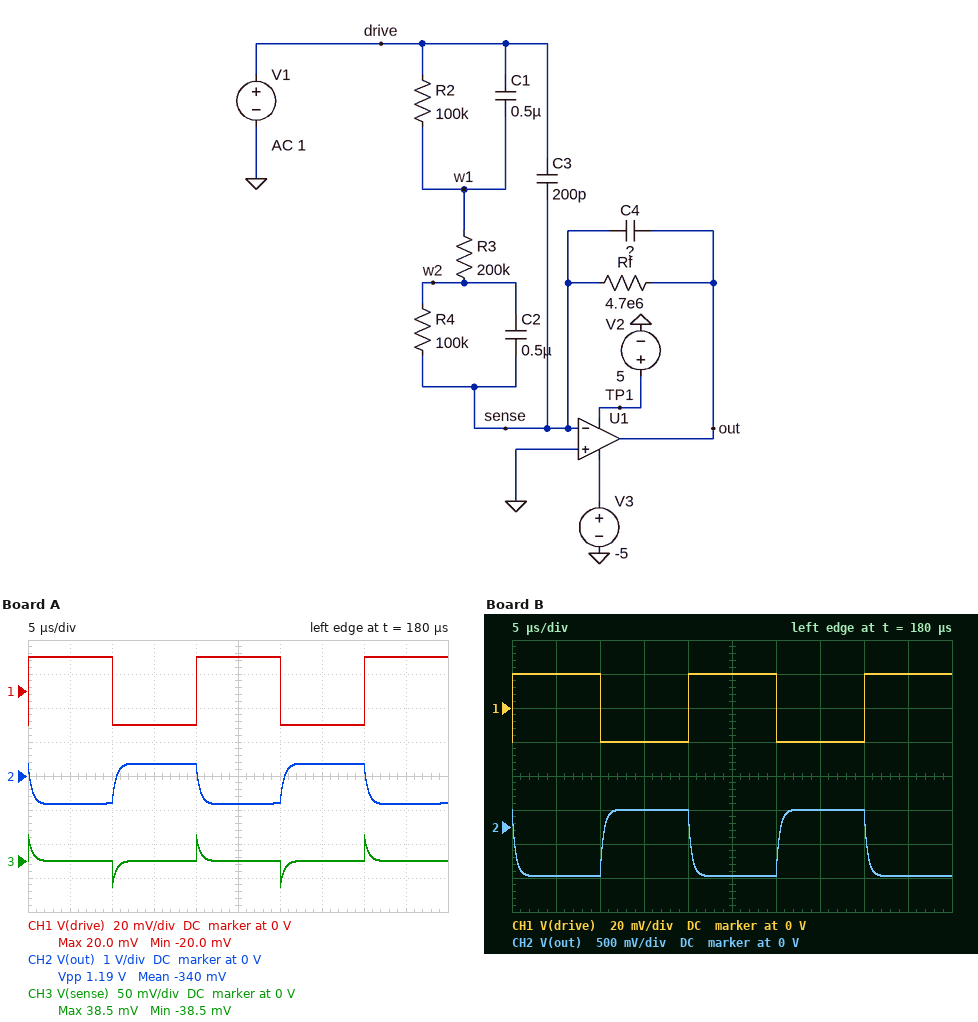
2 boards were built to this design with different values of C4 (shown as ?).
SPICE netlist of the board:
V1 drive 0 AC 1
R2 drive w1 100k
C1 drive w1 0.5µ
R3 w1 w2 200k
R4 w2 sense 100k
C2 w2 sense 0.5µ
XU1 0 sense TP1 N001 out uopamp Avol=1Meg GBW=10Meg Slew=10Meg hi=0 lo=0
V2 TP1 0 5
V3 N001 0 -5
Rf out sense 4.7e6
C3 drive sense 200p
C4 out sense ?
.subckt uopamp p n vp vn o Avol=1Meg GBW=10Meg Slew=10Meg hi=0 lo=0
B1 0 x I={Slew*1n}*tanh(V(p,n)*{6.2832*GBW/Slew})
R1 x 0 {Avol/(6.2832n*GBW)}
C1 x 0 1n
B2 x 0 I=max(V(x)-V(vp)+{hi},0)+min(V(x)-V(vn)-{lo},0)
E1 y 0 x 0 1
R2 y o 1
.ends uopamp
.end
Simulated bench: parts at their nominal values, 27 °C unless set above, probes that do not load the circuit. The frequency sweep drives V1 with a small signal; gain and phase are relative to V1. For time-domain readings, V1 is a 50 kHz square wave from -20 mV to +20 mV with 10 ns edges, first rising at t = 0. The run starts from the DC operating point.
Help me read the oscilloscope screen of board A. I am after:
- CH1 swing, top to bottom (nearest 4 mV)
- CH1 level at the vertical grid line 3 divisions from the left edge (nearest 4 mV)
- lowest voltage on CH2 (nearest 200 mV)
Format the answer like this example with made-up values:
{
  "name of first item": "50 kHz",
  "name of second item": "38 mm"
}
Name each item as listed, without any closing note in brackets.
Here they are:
{
  "CH1 swing, top to bottom": "40 mV",
  "CH1 level at the vertical grid line 3 divisions from the left edge": "-20 mV",
  "lowest voltage on CH2": "-800 mV"
}
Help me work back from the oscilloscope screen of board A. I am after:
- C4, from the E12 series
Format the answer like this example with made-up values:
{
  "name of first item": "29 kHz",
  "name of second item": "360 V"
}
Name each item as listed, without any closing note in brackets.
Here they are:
{
  "C4, from the E12 series": "6.8 pF"
}
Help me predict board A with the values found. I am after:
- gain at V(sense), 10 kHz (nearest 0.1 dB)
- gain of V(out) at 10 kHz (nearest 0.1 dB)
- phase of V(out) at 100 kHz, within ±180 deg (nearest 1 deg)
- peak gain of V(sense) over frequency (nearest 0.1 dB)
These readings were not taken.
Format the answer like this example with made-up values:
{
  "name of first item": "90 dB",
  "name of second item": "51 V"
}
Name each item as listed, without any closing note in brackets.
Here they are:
{
  "gain at V(sense), 10 kHz": "-30.9 dB",
  "gain of V(out) at 10 kHz": "29.1 dB",
  "phase of V(out) at 100 kHz, within ±180 deg": "164 deg",
  "peak gain of V(sense) over frequency": "-0.3 dB"
}
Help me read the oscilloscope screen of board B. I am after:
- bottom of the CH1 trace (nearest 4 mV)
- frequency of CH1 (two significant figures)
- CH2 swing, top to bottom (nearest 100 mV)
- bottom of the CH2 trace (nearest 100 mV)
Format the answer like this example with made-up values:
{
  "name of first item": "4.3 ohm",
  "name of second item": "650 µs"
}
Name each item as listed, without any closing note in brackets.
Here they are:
{
  "bottom of the CH1 trace": "-20 mV",
  "frequency of CH1": "50 kHz",
  "CH2 swing, top to bottom": "1.0 V",
  "bottom of the CH2 trace": "-700 mV"
}
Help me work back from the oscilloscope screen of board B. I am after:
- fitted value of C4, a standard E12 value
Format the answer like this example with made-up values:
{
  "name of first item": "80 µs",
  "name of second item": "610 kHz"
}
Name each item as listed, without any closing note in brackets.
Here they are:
{
  "fitted value of C4, a standard E12 value": "8.2 pF"
}
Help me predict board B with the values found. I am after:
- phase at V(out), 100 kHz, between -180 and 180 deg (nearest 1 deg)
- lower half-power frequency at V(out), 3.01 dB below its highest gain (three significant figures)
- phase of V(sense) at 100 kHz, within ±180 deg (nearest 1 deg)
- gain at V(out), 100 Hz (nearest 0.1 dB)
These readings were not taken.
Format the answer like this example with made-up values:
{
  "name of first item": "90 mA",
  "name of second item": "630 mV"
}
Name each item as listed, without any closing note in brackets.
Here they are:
{
  "phase at V(out), 100 kHz, between -180 and 180 deg": "166 deg",
  "lower half-power frequency at V(out), 3.01 dB below its highest gain": "4.99 Hz",
  "phase of V(sense) at 100 kHz, within ±180 deg": "76 deg",
  "gain at V(out), 100 Hz": "27.4 dB"
}
